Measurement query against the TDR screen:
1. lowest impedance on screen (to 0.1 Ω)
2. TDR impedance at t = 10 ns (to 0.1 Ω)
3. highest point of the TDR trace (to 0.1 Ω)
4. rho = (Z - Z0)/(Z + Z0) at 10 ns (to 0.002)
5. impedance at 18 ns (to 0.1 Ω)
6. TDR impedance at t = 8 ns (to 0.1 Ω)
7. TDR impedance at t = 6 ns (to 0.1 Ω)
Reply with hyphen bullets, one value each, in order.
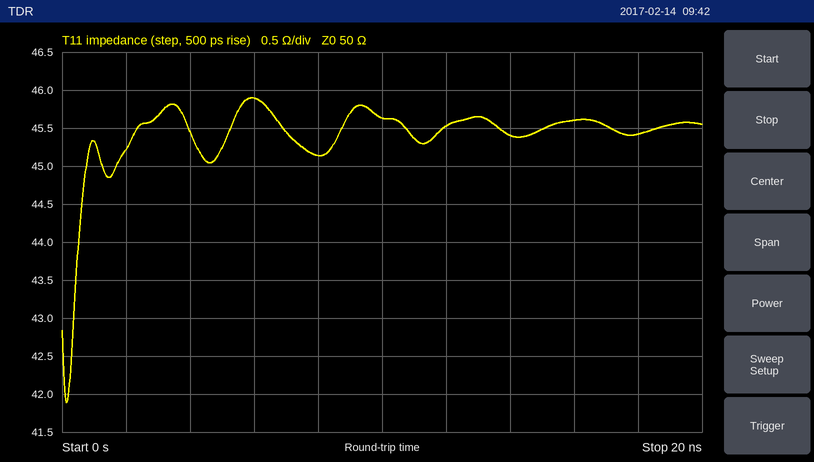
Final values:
- 41.9 Ω
- 45.6 Ω
- 45.9 Ω
- -0.046
- 45.4 Ω
- 45.1 Ω
- 45.9 Ω
